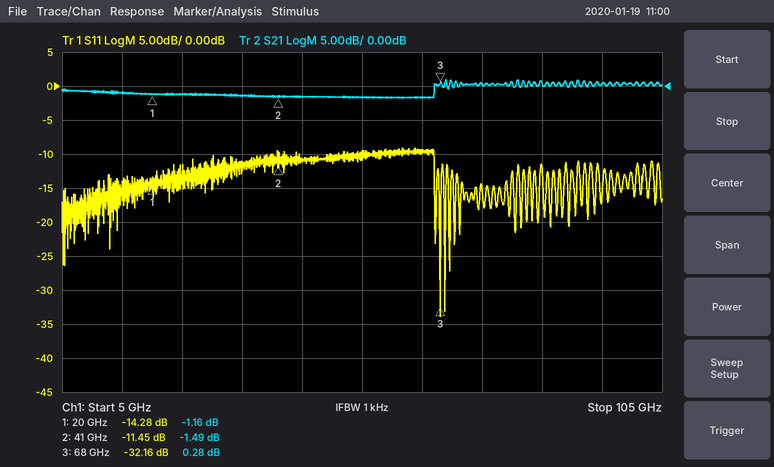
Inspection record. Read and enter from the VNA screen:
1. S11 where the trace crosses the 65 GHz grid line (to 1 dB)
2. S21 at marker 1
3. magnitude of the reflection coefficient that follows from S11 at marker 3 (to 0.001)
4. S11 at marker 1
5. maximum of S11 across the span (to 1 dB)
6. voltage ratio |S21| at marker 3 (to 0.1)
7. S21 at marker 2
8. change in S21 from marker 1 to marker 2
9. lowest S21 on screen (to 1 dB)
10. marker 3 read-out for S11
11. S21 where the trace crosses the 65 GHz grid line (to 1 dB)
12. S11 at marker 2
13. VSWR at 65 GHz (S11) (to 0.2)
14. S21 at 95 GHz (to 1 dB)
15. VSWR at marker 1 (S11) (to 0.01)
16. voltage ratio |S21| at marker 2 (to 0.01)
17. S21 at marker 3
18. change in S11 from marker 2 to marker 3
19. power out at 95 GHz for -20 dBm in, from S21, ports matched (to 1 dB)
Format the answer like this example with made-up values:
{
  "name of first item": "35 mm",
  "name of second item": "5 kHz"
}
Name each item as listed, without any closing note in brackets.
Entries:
{
  "S11 where the trace crosses the 65 GHz grid line": "-10 dB",
  "S21 at marker 1": "-1.16 dB",
  "magnitude of the reflection coefficient that follows from S11 at marker 3": "0.025",
  "S11 at marker 1": "-14.28 dB",
  "maximum of S11 across the span": "-9 dB",
  "voltage ratio |S21| at marker 3": "1.0",
  "S21 at marker 2": "-1.49 dB",
  "change in S21 from marker 1 to marker 2": "-0.33 dB",
  "lowest S21 on screen": "-2 dB",
  "marker 3 read-out for S11": "-32.16 dB",
  "S21 where the trace crosses the 65 GHz grid line": "-2 dB",
  "S11 at marker 2": "-11.45 dB",
  "VSWR at 65 GHz (S11)": "2.0",
  "S21 at 95 GHz": "0 dB",
  "VSWR at marker 1 (S11)": "1.48",
  "voltage ratio |S21| at marker 2": "0.84",
  "S21 at marker 3": "0.28 dB",
  "change in S11 from marker 2 to marker 3": "-20.71 dB",
  "power out at 95 GHz for -20 dBm in, from S21, ports matched": "-20 dBm"
}
